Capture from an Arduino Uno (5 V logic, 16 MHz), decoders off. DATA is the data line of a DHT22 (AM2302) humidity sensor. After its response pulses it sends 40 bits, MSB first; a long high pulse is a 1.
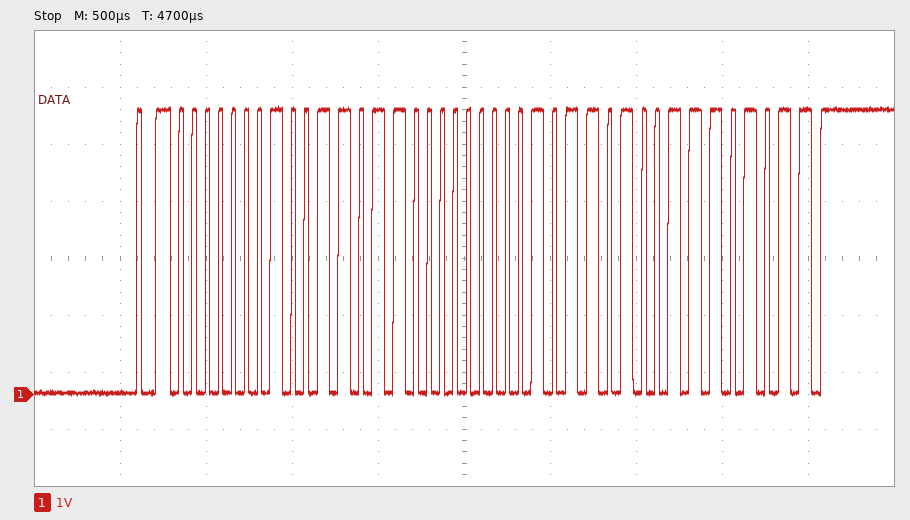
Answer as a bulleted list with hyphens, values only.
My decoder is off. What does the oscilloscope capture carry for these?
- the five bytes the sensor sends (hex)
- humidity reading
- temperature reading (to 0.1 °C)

- 01 36 00 B4 EB
- 31.0 %
- 18.0 °C
